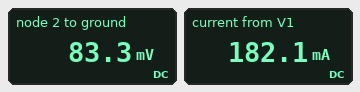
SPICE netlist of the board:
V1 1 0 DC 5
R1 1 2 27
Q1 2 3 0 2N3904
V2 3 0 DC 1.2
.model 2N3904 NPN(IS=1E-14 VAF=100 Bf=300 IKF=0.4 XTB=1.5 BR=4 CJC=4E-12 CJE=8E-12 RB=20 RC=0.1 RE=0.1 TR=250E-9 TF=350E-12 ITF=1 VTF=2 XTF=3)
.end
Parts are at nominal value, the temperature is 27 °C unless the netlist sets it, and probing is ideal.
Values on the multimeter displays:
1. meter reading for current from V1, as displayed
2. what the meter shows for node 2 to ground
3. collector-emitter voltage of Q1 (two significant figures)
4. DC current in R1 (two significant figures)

182.1 mA
83.3 mV
83 mV
180 mA
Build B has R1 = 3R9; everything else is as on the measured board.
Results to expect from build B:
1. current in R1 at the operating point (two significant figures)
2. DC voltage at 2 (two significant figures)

1.0 A
1.1 V
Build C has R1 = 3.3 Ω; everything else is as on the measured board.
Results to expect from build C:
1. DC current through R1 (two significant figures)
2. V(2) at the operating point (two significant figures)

1.0 A
1.7 V
